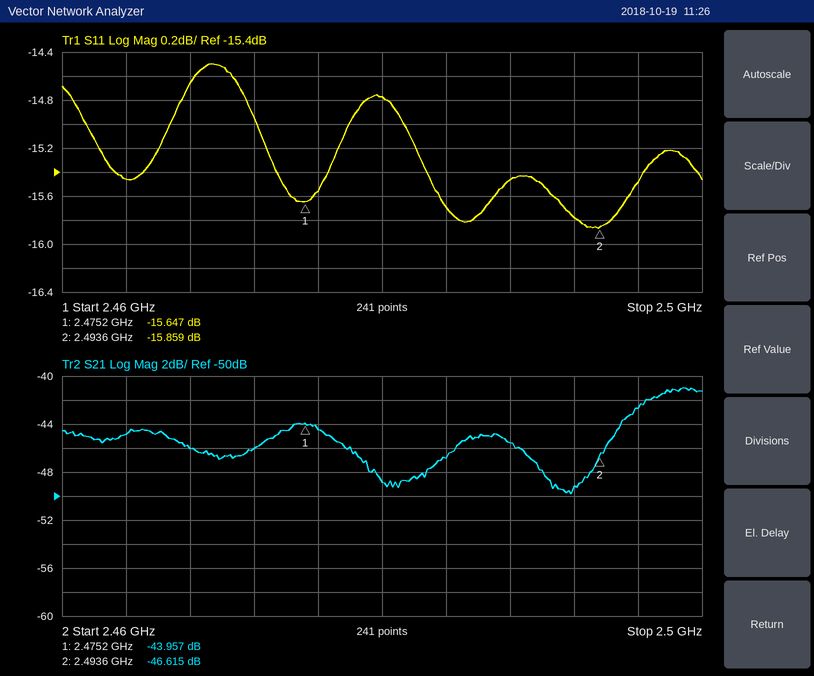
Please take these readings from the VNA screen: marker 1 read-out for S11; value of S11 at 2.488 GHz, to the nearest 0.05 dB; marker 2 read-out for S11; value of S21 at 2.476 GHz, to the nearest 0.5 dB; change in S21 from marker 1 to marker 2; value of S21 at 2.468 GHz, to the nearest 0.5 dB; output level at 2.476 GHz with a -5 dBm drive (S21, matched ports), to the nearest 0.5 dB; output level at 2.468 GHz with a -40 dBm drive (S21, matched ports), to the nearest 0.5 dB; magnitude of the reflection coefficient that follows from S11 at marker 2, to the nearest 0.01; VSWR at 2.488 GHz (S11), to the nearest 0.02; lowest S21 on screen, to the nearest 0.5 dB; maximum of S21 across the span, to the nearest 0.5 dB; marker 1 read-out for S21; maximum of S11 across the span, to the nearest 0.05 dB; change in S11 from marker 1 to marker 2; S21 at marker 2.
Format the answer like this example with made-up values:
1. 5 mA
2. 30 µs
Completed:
1. -15.647 dB
2. -15.45 dB
3. -15.859 dB
4. -44.5 dB
5. -2.658 dB
6. -46.0 dB
7. -49.5 dBm
8. -86.0 dBm
9. 0.16
10. 1.40
11. -50.0 dB
12. -41.0 dB
13. -43.957 dB
14. -14.50 dB
15. -0.212 dB
16. -46.615 dB
